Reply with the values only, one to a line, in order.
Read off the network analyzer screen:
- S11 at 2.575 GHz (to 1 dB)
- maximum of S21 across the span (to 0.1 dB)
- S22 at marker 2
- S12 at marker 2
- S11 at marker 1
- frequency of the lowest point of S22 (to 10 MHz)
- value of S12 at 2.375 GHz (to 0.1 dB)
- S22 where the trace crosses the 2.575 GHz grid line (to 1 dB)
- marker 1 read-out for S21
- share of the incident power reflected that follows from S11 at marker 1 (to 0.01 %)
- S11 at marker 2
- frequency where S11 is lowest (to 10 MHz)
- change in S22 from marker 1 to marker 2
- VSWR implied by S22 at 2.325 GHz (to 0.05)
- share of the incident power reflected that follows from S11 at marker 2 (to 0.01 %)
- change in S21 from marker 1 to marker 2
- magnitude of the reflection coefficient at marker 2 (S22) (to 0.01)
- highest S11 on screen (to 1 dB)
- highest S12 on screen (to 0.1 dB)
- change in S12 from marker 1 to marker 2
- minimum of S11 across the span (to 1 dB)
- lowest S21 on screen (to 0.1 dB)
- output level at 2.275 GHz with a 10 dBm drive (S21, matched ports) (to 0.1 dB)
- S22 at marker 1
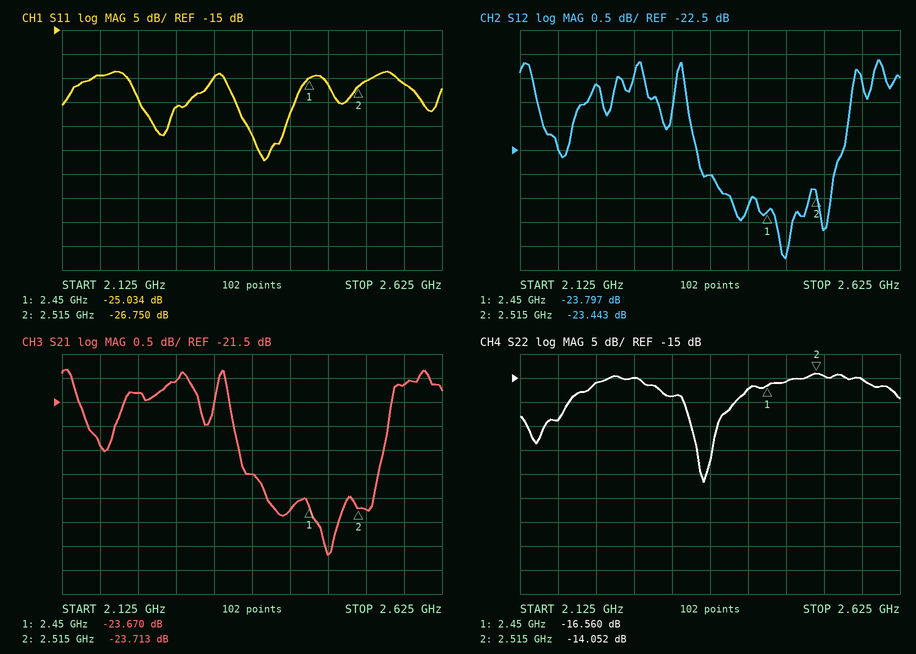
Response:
-26 dB
-20.8 dB
-14.052 dB
-23.443 dB
-25.034 dB
2.37 GHz
-23.0 dB
-15 dB
-23.670 dB
0.31 %
-26.750 dB
2.39 GHz
2.508 dB
1.25
0.21 %
-0.043 dB
0.20
-24 dB
-20.6 dB
0.354 dB
-42 dB
-24.7 dB
-11.1 dBm
-16.560 dB
